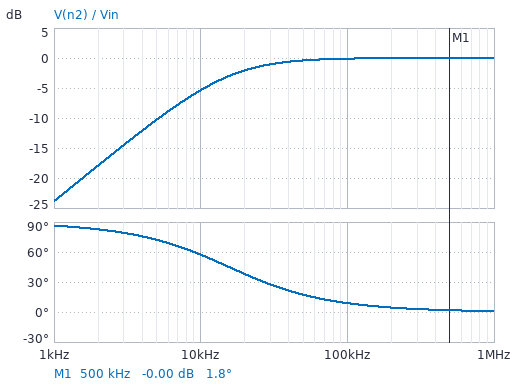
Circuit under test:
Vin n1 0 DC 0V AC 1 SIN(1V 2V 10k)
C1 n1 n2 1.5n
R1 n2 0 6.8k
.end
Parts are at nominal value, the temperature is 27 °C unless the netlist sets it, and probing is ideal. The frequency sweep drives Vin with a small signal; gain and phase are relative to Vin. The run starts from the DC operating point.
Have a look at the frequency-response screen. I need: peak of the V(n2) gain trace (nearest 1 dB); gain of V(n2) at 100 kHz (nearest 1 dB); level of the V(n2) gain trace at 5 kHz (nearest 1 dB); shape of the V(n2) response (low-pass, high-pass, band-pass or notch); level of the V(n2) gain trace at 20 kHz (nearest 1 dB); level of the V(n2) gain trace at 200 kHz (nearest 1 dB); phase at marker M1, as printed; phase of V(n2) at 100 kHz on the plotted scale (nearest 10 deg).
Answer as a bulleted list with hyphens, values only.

- 0 dB
- 0 dB
- -10 dB
- high-pass
- -2 dB
- 0 dB
- 1.8 deg
- 10 deg
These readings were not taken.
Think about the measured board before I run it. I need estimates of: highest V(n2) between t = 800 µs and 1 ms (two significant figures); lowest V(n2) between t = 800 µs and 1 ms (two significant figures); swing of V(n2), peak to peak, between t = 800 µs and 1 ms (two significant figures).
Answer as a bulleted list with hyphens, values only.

- 1.1 V
- -1.1 V
- 2.2 V
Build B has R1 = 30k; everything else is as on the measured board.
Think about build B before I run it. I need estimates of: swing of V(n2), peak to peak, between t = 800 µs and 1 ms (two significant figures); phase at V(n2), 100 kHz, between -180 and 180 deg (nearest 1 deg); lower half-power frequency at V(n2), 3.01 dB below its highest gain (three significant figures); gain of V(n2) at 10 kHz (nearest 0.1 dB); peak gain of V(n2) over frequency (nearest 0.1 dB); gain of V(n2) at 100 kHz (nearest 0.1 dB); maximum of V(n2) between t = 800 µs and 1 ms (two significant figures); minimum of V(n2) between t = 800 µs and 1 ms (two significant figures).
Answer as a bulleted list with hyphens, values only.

- 3.8 V
- 2 deg
- 3.54 kHz
- -0.5 dB
- 0 dB
- 0 dB
- 1.9 V
- -1.9 V
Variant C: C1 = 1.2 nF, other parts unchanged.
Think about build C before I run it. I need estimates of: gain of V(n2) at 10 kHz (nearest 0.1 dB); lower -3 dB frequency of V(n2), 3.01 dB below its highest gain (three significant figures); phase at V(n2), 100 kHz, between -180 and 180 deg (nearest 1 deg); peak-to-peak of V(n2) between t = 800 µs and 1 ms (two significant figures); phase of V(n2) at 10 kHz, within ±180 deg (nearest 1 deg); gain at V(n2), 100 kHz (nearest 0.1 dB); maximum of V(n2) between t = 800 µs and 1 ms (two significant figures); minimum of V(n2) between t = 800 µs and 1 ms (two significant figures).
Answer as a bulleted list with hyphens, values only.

- -6.8 dB
- 19.5 kHz
- 11 deg
- 1.8 V
- 63 deg
- -0.2 dB
- 910 mV
- -910 mV
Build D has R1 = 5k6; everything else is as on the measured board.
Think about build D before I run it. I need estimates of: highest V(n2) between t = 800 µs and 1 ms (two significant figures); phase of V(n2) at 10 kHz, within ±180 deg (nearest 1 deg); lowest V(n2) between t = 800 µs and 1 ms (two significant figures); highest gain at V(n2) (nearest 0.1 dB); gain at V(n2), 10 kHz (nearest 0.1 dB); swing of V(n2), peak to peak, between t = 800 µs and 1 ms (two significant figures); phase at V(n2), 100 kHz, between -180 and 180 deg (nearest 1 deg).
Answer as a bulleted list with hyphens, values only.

- 930 mV
- 62 deg
- -930 mV
- 0 dB
- -6.6 dB
- 1.9 V
- 11 deg
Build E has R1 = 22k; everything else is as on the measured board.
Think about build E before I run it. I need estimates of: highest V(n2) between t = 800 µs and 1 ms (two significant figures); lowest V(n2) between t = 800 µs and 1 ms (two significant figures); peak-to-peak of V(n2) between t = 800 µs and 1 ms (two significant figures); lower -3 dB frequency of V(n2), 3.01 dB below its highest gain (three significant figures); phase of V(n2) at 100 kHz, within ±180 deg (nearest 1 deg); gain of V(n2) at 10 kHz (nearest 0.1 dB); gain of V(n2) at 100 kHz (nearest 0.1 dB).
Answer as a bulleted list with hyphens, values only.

- 1.8 V
- -1.8 V
- 3.6 V
- 4.82 kHz
- 3 deg
- -0.9 dB
- 0 dB
